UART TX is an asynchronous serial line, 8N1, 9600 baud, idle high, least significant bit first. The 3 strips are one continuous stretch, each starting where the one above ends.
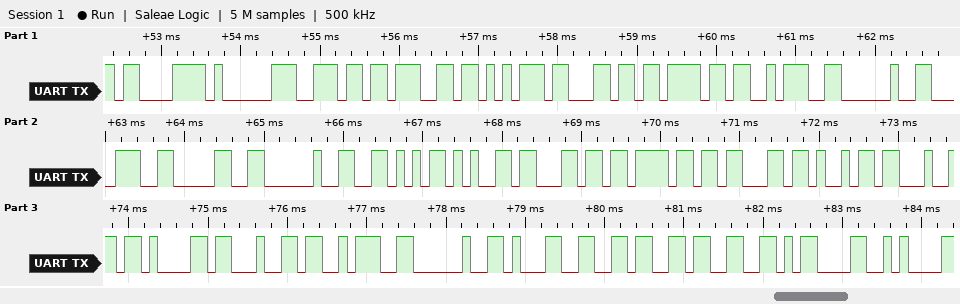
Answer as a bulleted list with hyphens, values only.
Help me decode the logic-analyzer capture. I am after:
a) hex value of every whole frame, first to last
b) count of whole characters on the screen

- C3 81 6E 67 75 6C 6F 3A 20 38 30 20 56 65 6C 6F 63 69 64 61 64 3A 20 31 36 33 0D 0A
- 28
